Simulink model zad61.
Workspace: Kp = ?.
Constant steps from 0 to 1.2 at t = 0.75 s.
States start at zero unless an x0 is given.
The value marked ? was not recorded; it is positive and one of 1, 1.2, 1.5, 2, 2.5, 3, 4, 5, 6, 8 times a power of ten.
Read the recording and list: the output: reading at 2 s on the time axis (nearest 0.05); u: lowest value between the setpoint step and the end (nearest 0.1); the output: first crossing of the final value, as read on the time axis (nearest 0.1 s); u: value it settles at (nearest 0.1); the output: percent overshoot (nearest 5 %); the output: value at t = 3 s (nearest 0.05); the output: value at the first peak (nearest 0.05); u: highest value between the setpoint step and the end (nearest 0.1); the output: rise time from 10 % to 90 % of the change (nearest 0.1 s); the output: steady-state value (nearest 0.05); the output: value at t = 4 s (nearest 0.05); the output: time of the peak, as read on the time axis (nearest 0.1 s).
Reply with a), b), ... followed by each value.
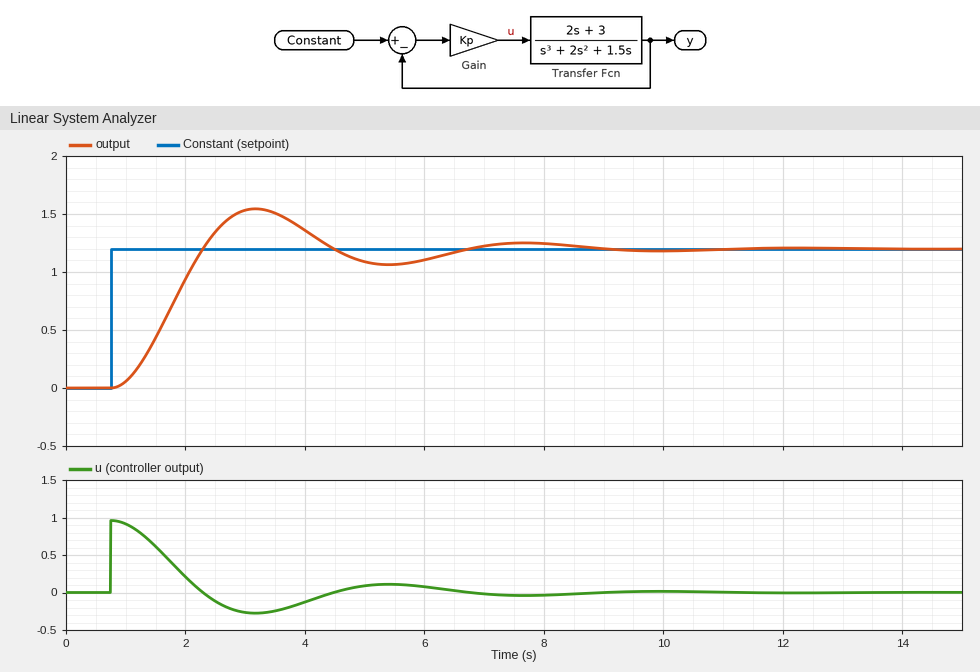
a) 0.95
b) -0.3
c) 2.3 s
d) 0.0
e) 30 %
f) 1.55
g) 1.55
h) 1.0
i) 1.0 s
j) 1.20
k) 1.35
l) 3.2 s
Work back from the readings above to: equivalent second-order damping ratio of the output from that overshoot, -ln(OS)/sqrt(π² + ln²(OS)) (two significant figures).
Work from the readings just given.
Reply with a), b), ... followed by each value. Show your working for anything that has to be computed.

a) ln(0.3) = -1.204; 1.204 / sqrt(9.870 + 1.450) = 0.36
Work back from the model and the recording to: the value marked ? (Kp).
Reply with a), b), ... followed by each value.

a) 0.8
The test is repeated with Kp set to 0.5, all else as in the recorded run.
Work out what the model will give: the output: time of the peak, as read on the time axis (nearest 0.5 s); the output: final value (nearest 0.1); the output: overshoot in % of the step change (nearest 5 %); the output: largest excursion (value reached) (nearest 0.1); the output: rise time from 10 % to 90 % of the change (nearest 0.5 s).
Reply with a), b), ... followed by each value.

a) 4.0 s
b) 1.2
c) 15 %
d) 1.4
e) 1.5 s
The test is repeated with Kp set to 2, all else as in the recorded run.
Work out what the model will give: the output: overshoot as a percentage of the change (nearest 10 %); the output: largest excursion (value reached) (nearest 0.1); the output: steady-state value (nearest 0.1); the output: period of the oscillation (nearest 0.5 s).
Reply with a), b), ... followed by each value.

a) 50 %
b) 1.8
c) 1.2
d) 3.0 s
